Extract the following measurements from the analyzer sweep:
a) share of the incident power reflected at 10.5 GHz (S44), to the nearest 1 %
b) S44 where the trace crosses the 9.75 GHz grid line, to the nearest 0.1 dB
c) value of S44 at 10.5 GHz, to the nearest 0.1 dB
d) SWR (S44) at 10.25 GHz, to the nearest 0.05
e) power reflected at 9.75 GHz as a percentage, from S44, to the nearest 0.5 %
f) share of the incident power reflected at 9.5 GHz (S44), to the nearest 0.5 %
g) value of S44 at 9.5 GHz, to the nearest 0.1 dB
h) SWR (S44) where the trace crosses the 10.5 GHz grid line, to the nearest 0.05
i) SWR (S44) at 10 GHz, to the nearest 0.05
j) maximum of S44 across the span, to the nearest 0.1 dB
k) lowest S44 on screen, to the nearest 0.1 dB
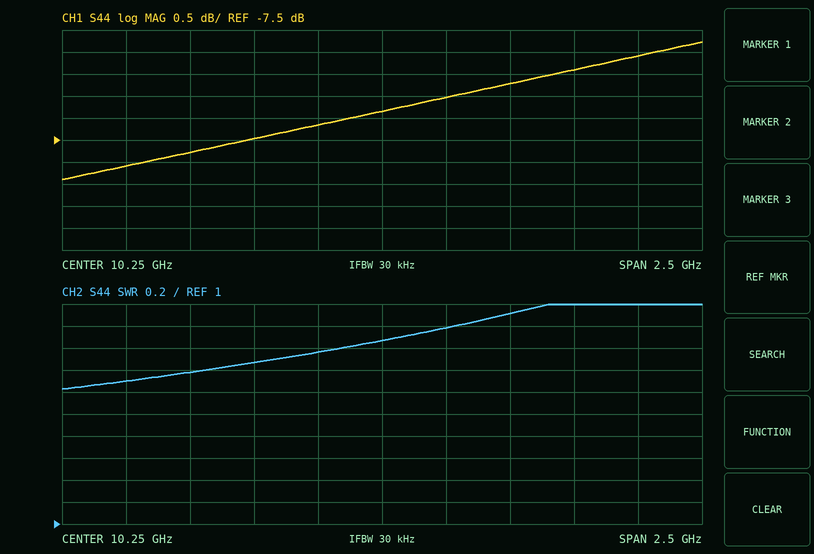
22 %
-7.5 dB
-6.5 dB
2.65
18.0 %
16.5 %
-7.8 dB
2.80
2.55
-5.3 dB
-8.4 dB
